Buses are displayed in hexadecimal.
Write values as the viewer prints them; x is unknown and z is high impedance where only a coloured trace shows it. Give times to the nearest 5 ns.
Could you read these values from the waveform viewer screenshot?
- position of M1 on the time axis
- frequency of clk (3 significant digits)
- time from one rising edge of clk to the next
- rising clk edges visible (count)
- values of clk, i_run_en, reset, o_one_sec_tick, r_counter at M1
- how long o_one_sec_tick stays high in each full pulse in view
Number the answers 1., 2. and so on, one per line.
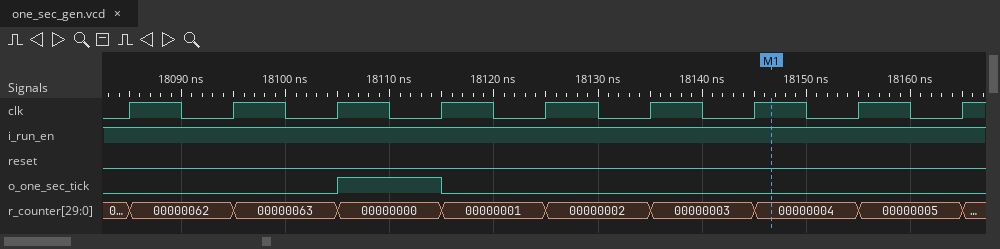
1. 18145 ns
2. 100 MHz
3. 10 ns
4. 9
5. clk=1, i_run_en=1, reset=0, o_one_sec_tick=0, r_counter=00000004
6. 10 ns
